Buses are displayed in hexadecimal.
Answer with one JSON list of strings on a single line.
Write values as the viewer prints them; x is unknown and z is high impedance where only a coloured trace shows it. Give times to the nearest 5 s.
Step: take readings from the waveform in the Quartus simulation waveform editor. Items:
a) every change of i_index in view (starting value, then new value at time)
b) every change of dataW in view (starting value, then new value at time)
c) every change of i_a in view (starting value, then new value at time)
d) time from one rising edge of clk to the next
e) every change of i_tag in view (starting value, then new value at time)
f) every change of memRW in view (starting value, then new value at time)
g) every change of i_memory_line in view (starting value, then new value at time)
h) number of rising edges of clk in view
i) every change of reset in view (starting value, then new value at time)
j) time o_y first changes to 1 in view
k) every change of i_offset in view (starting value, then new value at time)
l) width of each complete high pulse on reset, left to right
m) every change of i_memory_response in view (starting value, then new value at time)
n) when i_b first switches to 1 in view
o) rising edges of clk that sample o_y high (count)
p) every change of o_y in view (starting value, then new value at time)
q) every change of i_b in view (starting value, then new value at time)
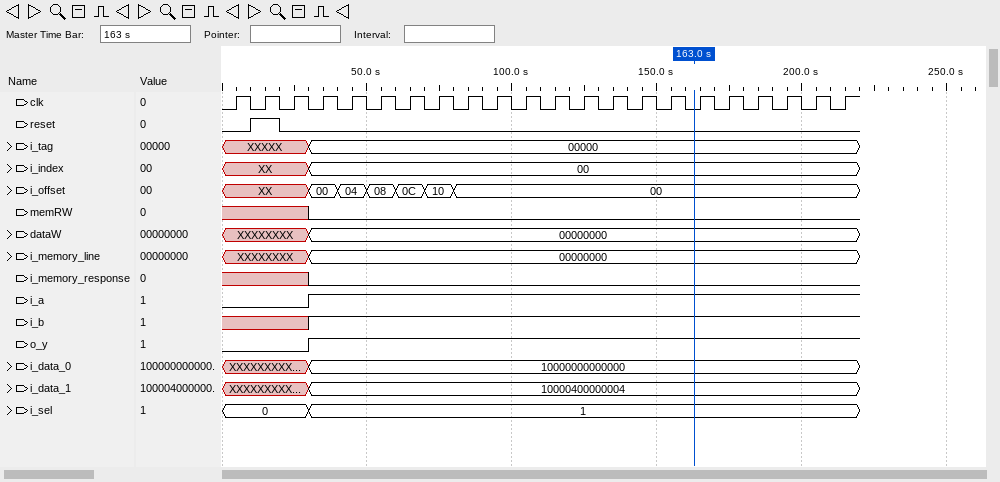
["XX, 00 at 30 s", "XXXXXXXX, 00000000 at 30 s", "0, 1 at 30 s", "10 s", "XXXXX, 00000 at 30 s", "x, 0 at 30 s", "XXXXXXXX, 00000000 at 30 s", "22", "0, 1 at 10 s, 0 at 20 s", "30 s", "XX, 00 at 30 s, 04 at 40 s, 08 at 50 s, 0C at 60 s, 10 at 70 s, 00 at 80 s", "10 s", "x, 0 at 30 s", "30 s", "19", "0, 1 at 30 s", "x, 1 at 30 s"]
